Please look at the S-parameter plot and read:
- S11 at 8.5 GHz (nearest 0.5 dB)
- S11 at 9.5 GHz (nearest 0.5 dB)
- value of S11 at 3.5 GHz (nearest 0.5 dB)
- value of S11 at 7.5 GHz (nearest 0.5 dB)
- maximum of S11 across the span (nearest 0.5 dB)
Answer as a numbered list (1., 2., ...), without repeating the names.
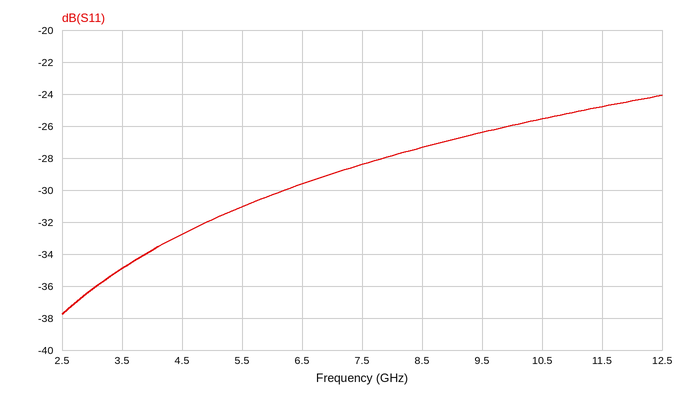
1. -27.5 dB
2. -26.5 dB
3. -35.0 dB
4. -28.5 dB
5. -24.0 dB
